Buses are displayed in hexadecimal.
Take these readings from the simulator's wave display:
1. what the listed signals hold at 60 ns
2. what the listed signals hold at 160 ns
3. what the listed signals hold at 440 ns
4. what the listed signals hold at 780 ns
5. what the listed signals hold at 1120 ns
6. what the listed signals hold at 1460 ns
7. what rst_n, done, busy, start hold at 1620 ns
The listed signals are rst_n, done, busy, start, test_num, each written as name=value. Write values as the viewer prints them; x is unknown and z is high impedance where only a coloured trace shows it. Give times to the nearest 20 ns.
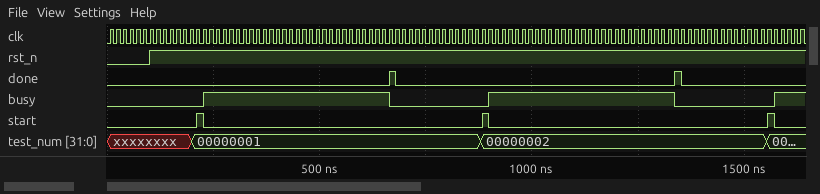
rst_n=0, done=0, busy=0, start=0, test_num=xxxxxxxx
rst_n=1, done=0, busy=0, start=0, test_num=xxxxxxxx
rst_n=1, done=0, busy=1, start=0, test_num=00000001
rst_n=1, done=0, busy=0, start=0, test_num=00000001
rst_n=1, done=0, busy=1, start=0, test_num=00000002
rst_n=1, done=0, busy=0, start=0, test_num=00000002
rst_n=1, done=0, busy=1, start=0
